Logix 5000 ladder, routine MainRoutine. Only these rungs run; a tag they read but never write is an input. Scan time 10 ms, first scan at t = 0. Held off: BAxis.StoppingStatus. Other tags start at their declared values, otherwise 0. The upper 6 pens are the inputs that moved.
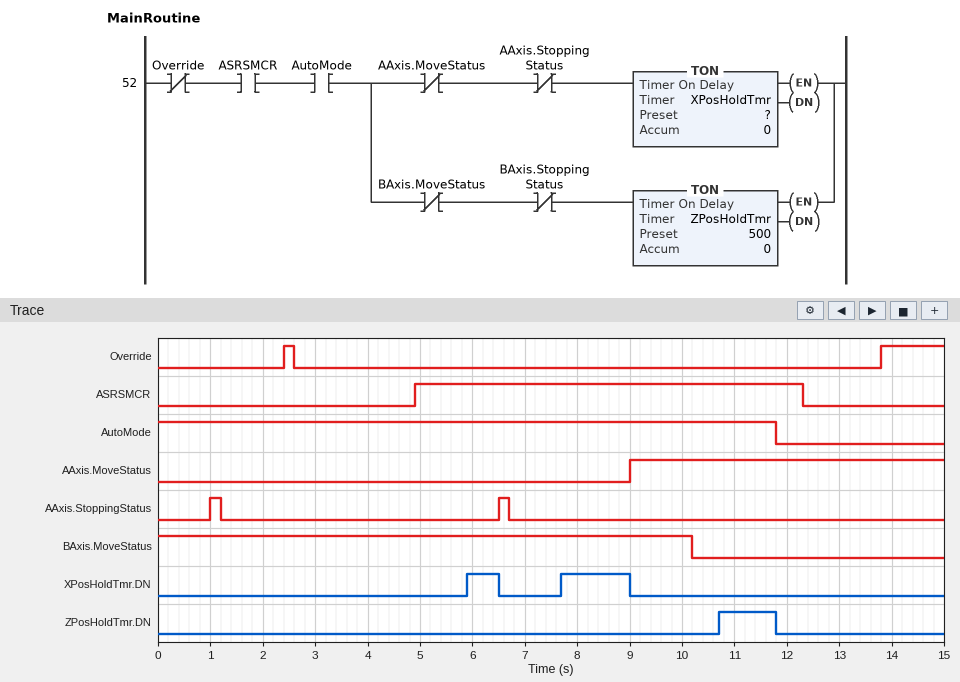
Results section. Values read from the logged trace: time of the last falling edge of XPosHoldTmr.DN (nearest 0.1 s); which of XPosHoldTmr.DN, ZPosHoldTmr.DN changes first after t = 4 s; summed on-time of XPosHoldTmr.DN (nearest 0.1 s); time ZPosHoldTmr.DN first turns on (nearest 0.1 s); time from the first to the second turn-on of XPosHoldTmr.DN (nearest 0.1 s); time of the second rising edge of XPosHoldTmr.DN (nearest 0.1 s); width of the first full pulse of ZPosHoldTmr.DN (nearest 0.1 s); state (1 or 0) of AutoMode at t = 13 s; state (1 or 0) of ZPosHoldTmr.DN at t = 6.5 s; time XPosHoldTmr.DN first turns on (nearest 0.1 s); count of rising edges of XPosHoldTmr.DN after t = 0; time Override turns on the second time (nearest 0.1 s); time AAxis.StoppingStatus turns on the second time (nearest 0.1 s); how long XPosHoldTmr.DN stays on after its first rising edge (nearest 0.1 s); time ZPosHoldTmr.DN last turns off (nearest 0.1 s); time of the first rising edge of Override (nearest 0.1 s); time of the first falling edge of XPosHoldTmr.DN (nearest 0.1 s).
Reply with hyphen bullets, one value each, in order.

- 9.0 s
- XPosHoldTmr.DN
- 1.9 s
- 10.7 s
- 1.8 s
- 7.7 s
- 1.1 s
- 0
- 0
- 5.9 s
- 2
- 13.8 s
- 6.5 s
- 0.6 s
- 11.8 s
- 2.4 s
- 6.5 s
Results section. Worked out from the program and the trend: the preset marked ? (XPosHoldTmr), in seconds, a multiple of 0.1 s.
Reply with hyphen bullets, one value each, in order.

- 1.0 s
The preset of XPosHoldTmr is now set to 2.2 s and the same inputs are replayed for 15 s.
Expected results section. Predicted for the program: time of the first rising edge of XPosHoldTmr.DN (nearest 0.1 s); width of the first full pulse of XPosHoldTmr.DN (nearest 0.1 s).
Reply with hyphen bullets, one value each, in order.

- 8.9 s
- 0.1 s
